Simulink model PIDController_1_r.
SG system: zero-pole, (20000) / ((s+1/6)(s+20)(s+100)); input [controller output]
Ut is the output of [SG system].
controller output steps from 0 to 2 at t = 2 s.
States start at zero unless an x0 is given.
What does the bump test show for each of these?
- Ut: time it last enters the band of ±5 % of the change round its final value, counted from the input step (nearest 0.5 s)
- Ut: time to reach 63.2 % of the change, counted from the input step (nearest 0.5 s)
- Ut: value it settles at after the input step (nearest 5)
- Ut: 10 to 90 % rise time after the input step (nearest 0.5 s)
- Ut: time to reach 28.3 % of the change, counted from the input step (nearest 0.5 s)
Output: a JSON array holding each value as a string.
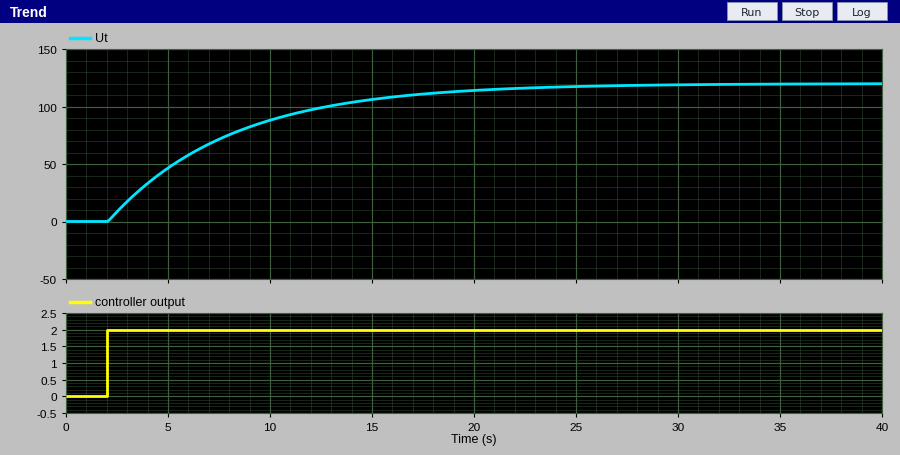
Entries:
["18.0 s", "6.0 s", "120", "13.0 s", "2.0 s"]
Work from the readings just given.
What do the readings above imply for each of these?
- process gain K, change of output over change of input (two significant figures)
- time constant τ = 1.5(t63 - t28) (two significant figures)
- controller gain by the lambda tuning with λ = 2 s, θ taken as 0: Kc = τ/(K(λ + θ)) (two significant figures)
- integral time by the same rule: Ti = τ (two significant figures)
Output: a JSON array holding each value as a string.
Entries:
["60", "6.0 s", "0.050", "6.0 s"]
